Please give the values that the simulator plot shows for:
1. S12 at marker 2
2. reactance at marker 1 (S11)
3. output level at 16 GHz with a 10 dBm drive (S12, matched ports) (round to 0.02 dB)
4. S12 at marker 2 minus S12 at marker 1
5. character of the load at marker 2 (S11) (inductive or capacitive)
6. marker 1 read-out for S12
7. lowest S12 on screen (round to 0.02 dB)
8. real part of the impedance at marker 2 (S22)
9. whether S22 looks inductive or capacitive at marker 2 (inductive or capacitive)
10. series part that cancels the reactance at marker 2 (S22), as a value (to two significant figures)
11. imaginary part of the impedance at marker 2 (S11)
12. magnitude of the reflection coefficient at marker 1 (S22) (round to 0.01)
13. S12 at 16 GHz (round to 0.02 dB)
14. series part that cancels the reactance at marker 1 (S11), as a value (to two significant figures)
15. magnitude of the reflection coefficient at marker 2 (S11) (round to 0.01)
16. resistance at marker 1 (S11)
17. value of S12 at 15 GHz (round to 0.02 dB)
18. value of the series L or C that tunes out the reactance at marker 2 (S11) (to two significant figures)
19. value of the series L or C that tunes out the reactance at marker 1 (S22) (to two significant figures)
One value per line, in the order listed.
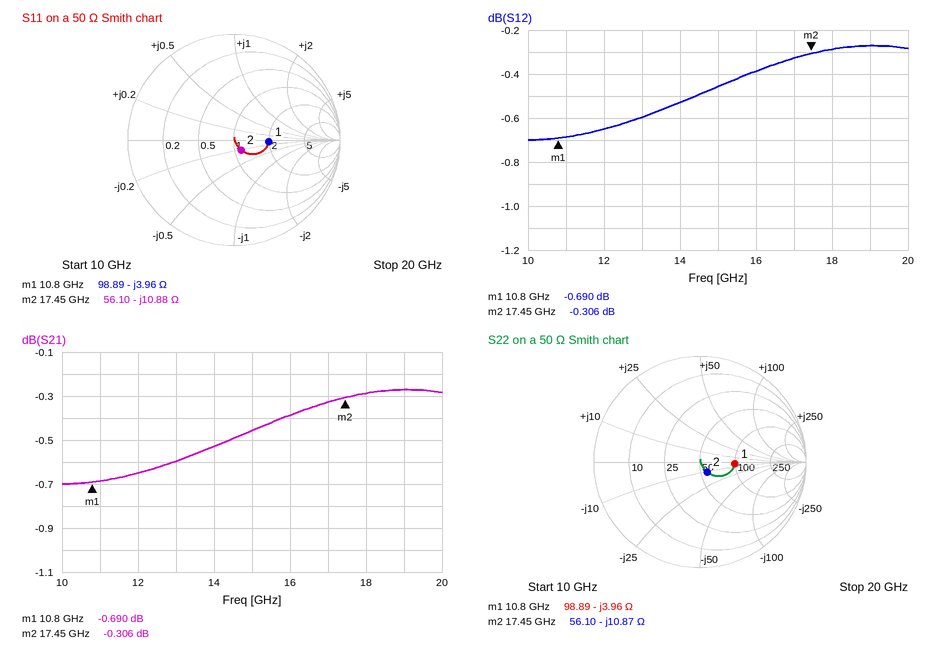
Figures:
-0.306 dB
-3.96 Ω
9.62 dBm
0.384 dB
capacitive
-0.690 dB
-0.70 dB
56.10 Ω
capacitive
99 pH
-10.88 Ω
0.33
-0.38 dB
58 pH
0.12
98.89 Ω
-0.46 dB
99 pH
58 pH
